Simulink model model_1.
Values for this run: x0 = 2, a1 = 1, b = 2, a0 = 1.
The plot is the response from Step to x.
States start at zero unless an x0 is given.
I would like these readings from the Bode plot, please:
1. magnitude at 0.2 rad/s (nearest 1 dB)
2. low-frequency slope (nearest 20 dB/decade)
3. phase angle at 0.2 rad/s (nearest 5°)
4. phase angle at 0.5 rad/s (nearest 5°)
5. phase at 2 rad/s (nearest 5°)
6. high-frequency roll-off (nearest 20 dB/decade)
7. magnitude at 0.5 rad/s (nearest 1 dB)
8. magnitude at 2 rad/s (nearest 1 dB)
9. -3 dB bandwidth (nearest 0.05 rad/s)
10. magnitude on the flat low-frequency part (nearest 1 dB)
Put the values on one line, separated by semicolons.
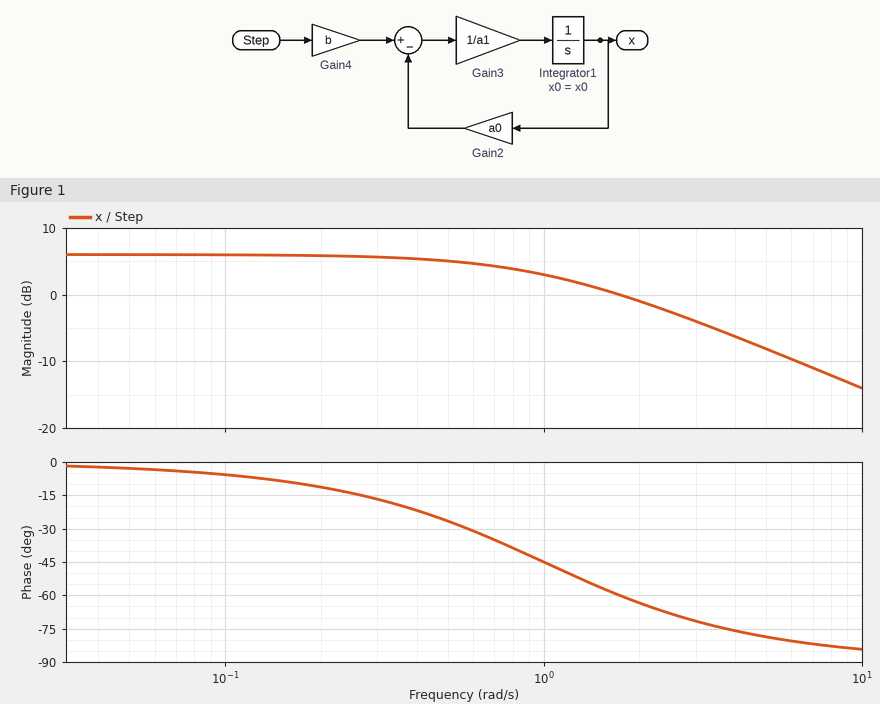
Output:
6 dB; 0 dB/decade; -10°; -25°; -65°; -20 dB/decade; 5 dB; -1 dB; 1.00 rad/s; 6 dB
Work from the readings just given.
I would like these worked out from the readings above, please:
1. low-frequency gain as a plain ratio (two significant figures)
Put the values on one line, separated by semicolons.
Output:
2.0
